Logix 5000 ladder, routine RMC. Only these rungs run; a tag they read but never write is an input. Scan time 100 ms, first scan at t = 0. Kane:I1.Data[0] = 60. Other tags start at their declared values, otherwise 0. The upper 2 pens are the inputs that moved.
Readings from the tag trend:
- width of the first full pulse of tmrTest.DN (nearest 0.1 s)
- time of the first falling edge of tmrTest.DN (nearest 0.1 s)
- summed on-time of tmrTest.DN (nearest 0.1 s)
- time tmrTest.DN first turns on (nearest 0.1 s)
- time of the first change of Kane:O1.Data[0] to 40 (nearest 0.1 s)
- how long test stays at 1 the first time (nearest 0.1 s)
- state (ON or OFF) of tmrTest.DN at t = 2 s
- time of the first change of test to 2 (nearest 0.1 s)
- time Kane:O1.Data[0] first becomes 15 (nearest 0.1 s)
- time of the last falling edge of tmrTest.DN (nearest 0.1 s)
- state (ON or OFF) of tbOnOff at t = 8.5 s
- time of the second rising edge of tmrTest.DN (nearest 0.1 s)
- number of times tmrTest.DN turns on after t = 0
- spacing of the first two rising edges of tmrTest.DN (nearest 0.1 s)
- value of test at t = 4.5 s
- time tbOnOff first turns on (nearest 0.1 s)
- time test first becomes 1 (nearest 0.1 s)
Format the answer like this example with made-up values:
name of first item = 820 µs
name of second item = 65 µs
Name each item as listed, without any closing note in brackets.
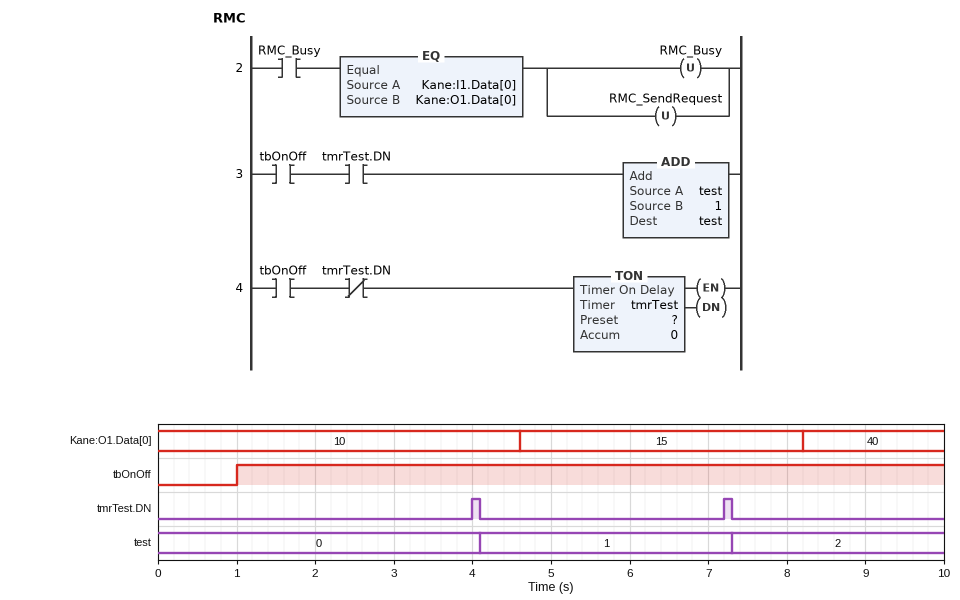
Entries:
width of the first full pulse of tmrTest.DN = 0.1 s
time of the first falling edge of tmrTest.DN = 4.1 s
summed on-time of tmrTest.DN = 0.2 s
time tmrTest.DN first turns on = 4.0 s
time of the first change of Kane:O1.Data[0] to 40 = 8.2 s
how long test stays at 1 the first time = 3.2 s
state (ON or OFF) of tmrTest.DN at t = 2 s = OFF
time of the first change of test to 2 = 7.3 s
time Kane:O1.Data[0] first becomes 15 = 4.6 s
time of the last falling edge of tmrTest.DN = 7.3 s
state (ON or OFF) of tbOnOff at t = 8.5 s = ON
time of the second rising edge of tmrTest.DN = 7.2 s
number of times tmrTest.DN turns on after t = 0 = 2
spacing of the first two rising edges of tmrTest.DN = 3.2 s
value of test at t = 4.5 s = 1
time tbOnOff first turns on = 1.0 s
time test first becomes 1 = 4.1 s
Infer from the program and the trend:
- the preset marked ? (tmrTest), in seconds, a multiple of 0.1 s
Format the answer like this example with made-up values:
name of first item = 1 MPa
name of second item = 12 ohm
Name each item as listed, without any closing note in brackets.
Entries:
the preset marked ? (tmrTest), in seconds, a multiple of 0.1 s = 3.0 s
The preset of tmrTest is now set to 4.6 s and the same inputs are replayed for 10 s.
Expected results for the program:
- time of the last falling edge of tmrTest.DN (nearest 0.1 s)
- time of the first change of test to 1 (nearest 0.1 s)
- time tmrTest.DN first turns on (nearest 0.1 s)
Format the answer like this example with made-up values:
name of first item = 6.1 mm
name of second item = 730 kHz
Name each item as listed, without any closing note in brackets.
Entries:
time of the last falling edge of tmrTest.DN = 5.7 s
time of the first change of test to 1 = 5.7 s
time tmrTest.DN first turns on = 5.6 s
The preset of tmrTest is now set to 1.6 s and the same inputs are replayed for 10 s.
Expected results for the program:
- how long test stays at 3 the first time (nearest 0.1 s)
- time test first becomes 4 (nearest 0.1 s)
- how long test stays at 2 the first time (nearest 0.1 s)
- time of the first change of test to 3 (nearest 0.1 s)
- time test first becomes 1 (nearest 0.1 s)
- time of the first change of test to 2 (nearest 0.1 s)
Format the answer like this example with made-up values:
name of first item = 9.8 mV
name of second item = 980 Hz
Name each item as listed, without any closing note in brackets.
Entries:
how long test stays at 3 the first time = 1.8 s
time test first becomes 4 = 8.1 s
how long test stays at 2 the first time = 1.8 s
time of the first change of test to 3 = 6.3 s
time test first becomes 1 = 2.7 s
time of the first change of test to 2 = 4.5 s
